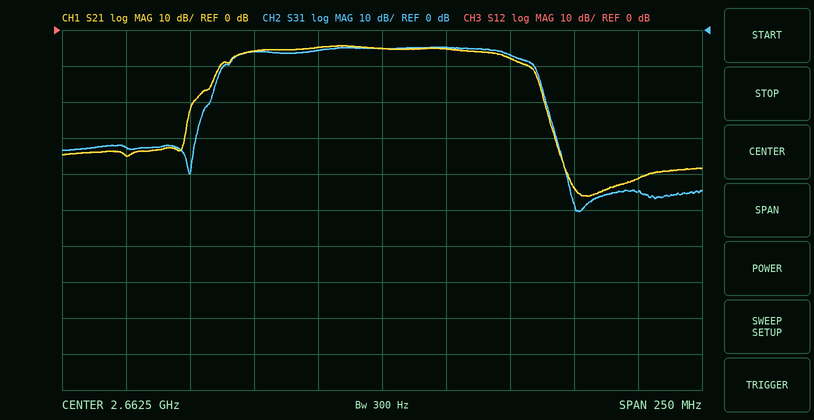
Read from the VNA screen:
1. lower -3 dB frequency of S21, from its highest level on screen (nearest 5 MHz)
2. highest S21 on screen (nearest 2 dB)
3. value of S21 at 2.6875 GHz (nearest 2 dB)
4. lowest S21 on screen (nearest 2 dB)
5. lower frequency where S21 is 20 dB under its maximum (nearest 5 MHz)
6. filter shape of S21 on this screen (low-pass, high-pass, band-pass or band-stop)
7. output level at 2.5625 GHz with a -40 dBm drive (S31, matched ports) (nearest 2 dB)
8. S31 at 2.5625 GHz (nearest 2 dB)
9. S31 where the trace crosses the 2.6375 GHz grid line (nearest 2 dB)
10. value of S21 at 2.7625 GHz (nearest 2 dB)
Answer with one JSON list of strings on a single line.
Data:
["2.605 GHz", "-4 dB", "-6 dB", "-46 dB", "2.585 GHz", "band-pass", "-72 dBm", "-32 dB", "-6 dB", "-42 dB"]
